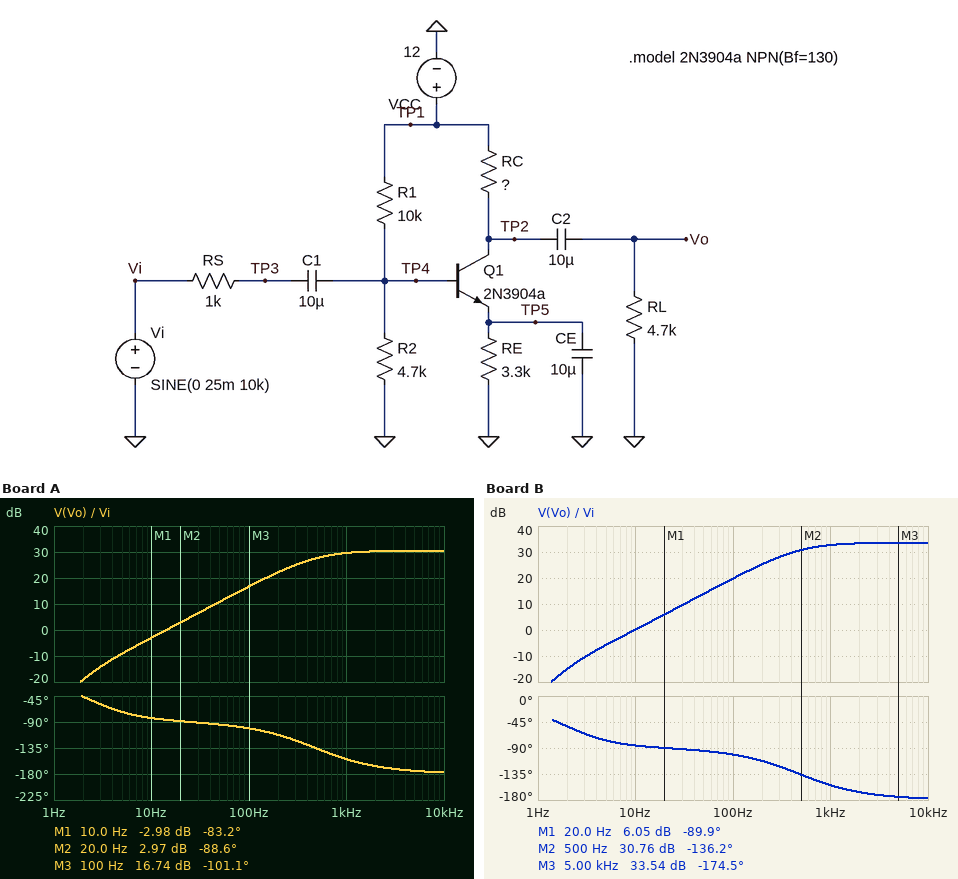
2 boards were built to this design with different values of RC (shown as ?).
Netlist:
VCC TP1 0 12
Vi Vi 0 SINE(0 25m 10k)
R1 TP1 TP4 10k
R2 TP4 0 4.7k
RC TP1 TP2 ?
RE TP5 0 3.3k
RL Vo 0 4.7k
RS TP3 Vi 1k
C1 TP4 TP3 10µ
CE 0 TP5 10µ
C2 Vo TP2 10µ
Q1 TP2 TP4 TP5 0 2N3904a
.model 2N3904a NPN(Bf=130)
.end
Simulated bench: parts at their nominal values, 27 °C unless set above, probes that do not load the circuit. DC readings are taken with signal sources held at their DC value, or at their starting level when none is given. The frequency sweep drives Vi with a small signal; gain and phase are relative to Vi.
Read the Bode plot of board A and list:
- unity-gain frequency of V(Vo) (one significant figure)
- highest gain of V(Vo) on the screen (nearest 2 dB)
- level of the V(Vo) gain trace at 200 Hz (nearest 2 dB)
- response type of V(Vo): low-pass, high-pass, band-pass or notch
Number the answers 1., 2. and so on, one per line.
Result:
1. 10 Hz
2. 30 dB
3. 22 dB
4. high-pass
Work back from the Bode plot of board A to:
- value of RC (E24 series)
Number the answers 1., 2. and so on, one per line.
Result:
1. 2.2 kΩ
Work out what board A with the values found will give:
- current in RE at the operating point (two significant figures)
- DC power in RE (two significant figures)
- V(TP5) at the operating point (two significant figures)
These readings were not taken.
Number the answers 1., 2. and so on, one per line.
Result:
1. 920 µA
2. 2.8 mW
3. 3.0 V
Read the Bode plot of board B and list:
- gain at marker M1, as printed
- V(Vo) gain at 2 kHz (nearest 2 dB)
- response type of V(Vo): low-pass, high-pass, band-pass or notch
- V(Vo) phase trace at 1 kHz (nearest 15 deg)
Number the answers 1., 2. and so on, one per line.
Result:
1. 6.05 dB
2. 34 dB
3. high-pass
4. -150 deg
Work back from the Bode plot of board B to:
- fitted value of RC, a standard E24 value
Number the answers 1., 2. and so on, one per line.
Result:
1. 3.9 kΩ
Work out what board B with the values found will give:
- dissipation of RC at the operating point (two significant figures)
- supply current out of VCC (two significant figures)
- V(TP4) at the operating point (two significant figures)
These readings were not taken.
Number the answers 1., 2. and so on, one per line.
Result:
1. 3.3 mW
2. 1.7 mA
3. 3.8 V
